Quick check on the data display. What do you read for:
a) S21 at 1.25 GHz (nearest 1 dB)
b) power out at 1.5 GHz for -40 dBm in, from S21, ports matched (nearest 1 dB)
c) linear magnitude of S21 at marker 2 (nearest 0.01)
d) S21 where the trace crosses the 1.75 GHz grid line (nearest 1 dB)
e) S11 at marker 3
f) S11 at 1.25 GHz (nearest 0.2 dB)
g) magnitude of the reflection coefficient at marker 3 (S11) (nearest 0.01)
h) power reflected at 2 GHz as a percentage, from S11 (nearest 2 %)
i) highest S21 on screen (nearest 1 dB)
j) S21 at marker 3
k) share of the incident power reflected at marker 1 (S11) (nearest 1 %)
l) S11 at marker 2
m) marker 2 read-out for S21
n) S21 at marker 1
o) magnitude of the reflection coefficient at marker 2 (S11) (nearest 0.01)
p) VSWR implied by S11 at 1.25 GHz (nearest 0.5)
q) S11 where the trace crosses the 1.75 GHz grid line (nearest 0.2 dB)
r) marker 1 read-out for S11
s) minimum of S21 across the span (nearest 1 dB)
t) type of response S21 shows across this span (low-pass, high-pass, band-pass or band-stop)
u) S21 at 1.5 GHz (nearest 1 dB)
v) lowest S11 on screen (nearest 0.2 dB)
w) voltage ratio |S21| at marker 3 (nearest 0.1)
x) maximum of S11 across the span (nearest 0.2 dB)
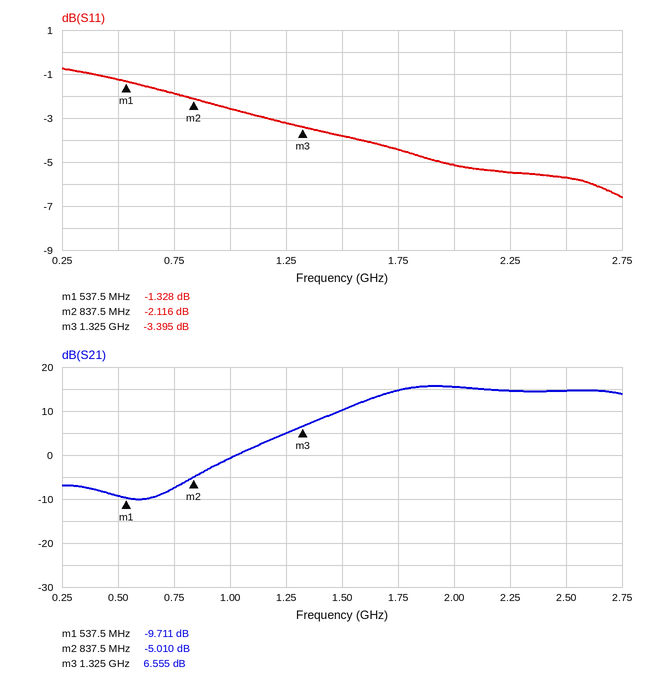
5 dB
-30 dBm
0.56
15 dB
-3.395 dB
-3.2 dB
0.68
30 %
16 dB
6.555 dB
74 %
-2.116 dB
-5.010 dB
-9.711 dB
0.78
5.5
-4.4 dB
-1.328 dB
-10 dB
high-pass
10 dB
-6.6 dB
2.1
-0.8 dB
